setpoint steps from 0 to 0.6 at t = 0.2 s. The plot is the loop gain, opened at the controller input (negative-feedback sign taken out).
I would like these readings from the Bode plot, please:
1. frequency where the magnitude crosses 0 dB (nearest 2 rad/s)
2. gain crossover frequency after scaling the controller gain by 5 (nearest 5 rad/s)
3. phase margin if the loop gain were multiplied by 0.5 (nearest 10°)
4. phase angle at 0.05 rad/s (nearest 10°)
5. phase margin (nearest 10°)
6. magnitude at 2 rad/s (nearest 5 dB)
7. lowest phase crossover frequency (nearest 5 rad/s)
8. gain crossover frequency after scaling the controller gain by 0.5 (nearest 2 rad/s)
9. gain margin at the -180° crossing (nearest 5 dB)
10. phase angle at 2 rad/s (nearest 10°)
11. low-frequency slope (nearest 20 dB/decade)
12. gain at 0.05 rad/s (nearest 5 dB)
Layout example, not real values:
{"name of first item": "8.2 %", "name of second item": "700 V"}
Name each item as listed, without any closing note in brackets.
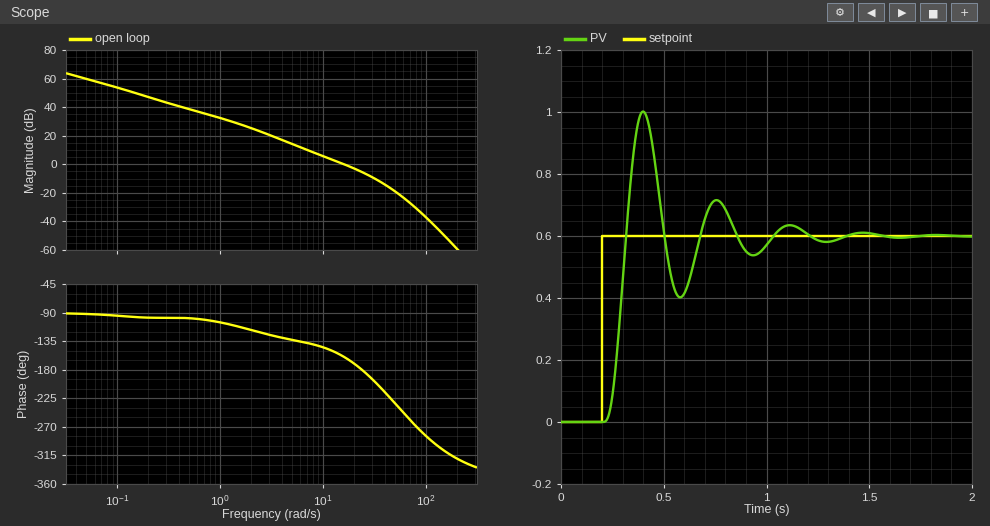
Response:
{"frequency where the magnitude crosses 0 dB": "16 rad/s", "gain crossover frequency after scaling the controller gain by 5": "40 rad/s", "phase margin if the loop gain were multiplied by 0.5": "40°", "phase angle at 0.05 rad/s": "-90°", "phase margin": "20°", "magnitude at 2 rad/s": "25 dB", "lowest phase crossover frequency": "25 rad/s", "gain crossover frequency after scaling the controller gain by 0.5": "10 rad/s", "gain margin at the -180° crossing": "5 dB", "phase angle at 2 rad/s": "-120°", "low-frequency slope": "-20 dB/decade", "gain at 0.05 rad/s": "60 dB"}
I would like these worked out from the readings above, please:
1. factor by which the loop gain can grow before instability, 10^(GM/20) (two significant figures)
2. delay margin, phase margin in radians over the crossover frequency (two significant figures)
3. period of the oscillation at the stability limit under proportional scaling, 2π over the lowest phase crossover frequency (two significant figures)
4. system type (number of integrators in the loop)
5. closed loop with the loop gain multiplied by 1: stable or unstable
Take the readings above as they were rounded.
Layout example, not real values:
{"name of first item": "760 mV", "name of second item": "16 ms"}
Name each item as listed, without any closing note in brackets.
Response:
{"factor by which the loop gain can grow before instability, 10^(GM/20)": "1.8", "delay margin, phase margin in radians over the crossover frequency": "0.022 s", "period of the oscillation at the stability limit under proportional scaling, 2π over the lowest phase crossover frequency": "0.25 s", "system type": "1", "closed loop with the loop gain multiplied by 1: stable or unstable": "stable"}
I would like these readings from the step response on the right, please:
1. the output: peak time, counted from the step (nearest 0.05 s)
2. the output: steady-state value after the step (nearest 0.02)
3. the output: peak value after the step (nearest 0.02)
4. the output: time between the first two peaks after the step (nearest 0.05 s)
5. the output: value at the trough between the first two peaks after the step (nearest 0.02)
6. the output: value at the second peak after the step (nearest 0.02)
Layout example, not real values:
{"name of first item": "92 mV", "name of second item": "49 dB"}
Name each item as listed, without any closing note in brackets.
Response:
{"the output: peak time, counted from the step": "0.20 s", "the output: steady-state value after the step": "0.60", "the output: peak value after the step": "1.00", "the output: time between the first two peaks after the step": "0.35 s", "the output: value at the trough between the first two peaks after the step": "0.40", "the output: value at the second peak after the step": "0.72"}
